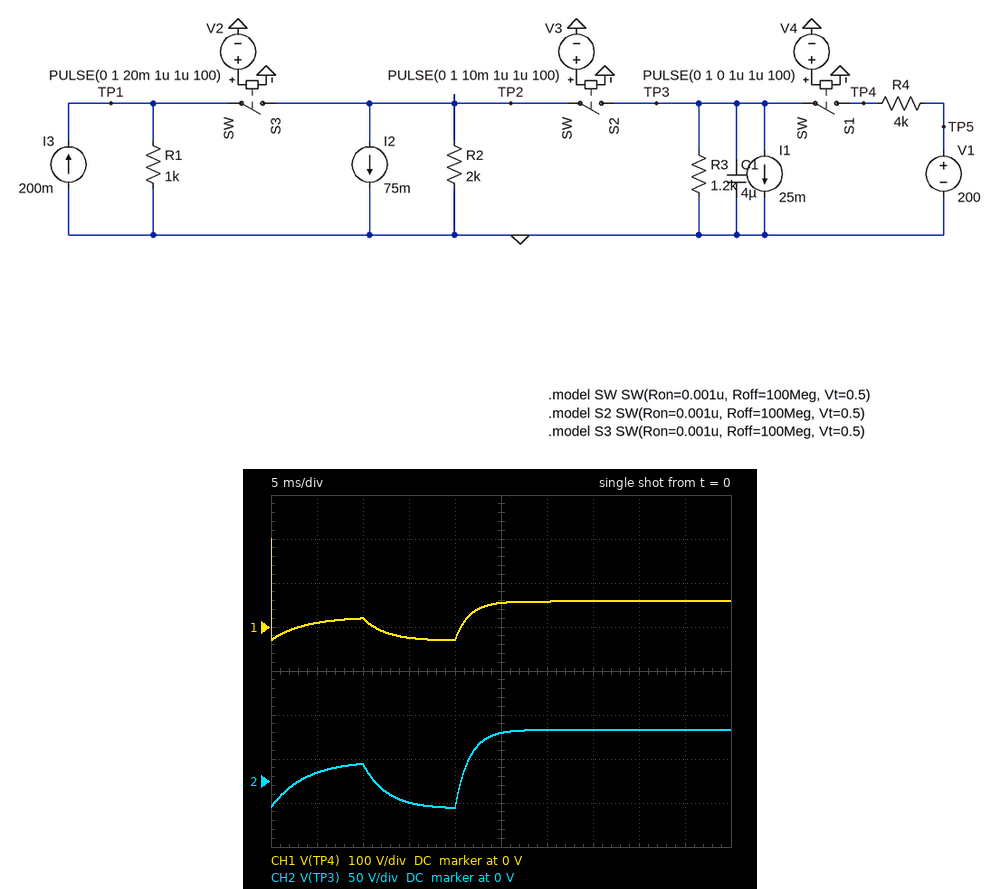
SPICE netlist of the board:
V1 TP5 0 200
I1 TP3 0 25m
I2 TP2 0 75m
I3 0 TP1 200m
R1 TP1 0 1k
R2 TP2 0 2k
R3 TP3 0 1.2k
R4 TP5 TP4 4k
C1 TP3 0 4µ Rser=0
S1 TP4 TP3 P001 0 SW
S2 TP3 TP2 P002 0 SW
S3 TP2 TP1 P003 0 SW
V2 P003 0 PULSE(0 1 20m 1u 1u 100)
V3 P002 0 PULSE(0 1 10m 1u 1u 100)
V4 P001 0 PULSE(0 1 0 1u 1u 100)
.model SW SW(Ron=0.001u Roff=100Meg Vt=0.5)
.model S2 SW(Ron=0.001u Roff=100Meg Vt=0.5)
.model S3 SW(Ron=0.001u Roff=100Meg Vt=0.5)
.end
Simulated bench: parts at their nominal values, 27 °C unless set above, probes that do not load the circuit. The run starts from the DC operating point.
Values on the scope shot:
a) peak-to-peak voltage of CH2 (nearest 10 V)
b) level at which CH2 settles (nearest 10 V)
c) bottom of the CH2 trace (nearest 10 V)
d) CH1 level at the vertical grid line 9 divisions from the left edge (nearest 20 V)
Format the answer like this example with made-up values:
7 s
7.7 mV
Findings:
90 V
60 V
-30 V
60 V
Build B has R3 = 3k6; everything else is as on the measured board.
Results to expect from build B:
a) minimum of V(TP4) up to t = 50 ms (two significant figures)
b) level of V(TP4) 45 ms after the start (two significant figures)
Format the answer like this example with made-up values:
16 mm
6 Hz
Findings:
-90 V
74 V
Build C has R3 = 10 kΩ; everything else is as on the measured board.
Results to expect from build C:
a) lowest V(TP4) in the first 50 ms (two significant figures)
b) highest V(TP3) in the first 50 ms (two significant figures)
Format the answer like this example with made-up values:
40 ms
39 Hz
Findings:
-250 V
81 V
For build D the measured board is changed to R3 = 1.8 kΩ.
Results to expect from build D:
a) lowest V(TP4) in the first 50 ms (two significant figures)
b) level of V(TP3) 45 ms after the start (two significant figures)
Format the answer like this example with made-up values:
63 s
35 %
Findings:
-45 V
65 V
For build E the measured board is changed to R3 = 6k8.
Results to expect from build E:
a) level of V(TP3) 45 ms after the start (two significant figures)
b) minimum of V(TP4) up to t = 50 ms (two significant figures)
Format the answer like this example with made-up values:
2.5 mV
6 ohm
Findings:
79 V
-170 V
